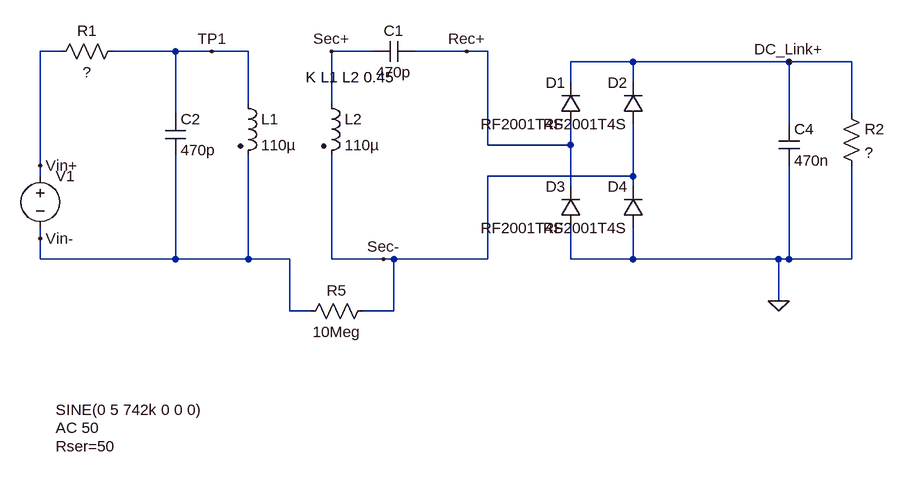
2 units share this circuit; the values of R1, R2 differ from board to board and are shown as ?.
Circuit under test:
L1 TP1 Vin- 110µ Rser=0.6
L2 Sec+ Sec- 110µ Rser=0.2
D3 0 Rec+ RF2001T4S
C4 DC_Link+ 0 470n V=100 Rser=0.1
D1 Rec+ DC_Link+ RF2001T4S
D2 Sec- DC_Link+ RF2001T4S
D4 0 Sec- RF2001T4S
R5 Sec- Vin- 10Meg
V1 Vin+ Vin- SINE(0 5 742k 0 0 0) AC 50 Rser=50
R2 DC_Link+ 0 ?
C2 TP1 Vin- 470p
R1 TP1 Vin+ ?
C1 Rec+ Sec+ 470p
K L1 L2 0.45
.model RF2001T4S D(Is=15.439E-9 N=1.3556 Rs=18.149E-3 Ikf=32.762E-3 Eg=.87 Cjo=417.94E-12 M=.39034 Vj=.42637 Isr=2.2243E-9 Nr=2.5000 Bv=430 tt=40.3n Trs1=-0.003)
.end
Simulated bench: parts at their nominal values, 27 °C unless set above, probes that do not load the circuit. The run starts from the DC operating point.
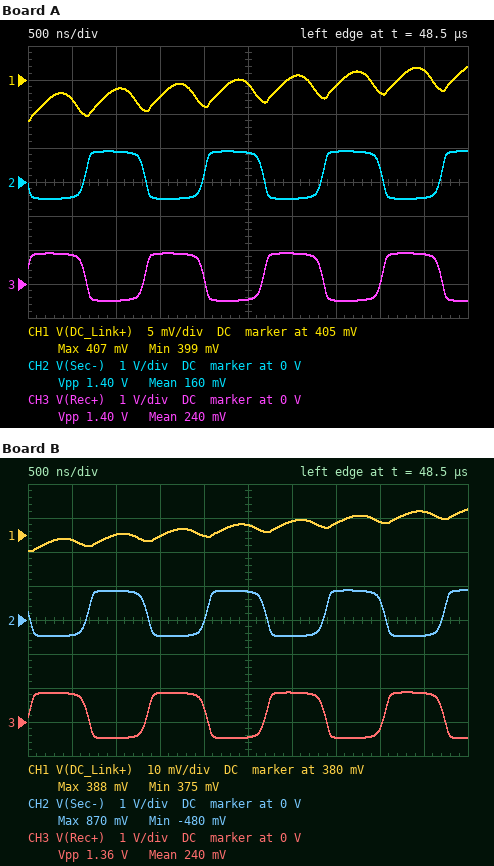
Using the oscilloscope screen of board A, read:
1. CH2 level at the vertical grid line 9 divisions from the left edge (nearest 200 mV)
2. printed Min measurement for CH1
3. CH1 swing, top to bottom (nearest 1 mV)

-400 mV
399 mV
8 mV
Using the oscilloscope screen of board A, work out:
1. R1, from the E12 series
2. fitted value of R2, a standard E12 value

39 Ω
68 Ω
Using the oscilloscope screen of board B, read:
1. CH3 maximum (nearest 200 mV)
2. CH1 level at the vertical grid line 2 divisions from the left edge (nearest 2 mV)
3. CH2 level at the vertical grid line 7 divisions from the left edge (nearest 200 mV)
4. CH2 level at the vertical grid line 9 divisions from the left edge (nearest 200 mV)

800 mV
380 mV
800 mV
-400 mV
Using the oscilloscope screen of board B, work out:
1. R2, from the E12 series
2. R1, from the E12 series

100 Ω
150 Ω
